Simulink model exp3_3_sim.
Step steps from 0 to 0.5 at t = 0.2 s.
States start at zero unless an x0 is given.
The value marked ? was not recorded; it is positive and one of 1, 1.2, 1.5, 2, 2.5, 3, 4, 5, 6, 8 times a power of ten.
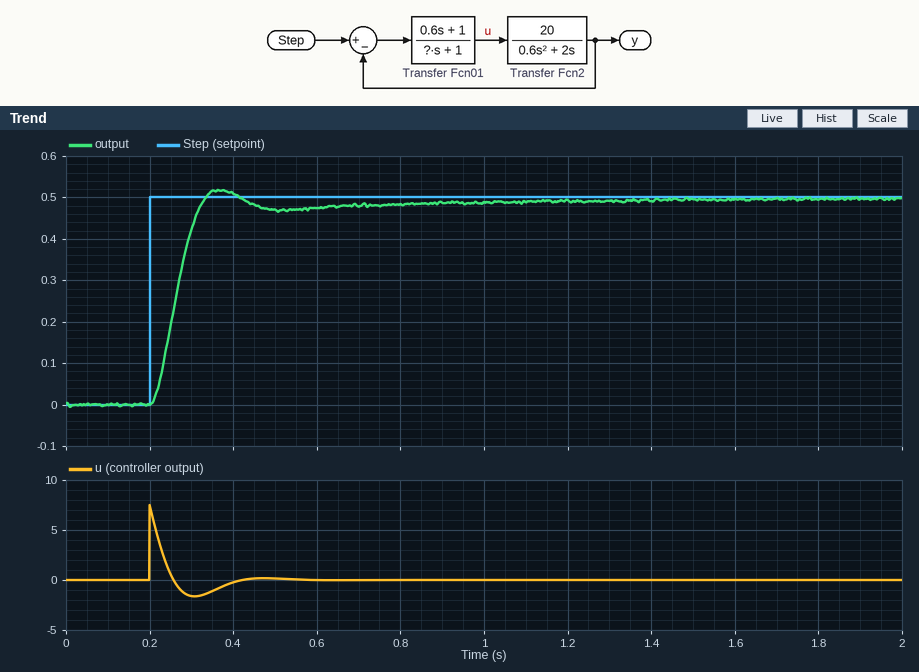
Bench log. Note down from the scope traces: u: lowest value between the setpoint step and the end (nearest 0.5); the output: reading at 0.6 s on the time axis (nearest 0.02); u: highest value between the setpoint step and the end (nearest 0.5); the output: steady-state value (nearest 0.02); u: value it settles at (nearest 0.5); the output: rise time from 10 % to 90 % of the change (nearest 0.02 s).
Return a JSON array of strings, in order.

["-1.5", "0.48", "7.5", "0.50", "0.0", "0.08 s"]
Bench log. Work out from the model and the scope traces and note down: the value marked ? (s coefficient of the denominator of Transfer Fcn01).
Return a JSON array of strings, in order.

["0.04"]
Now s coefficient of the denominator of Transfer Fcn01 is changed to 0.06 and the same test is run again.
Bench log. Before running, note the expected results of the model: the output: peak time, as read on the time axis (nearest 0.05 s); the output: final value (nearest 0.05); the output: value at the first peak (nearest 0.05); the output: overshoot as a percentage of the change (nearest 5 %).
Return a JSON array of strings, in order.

["0.40 s", "0.50", "0.55", "10 %"]
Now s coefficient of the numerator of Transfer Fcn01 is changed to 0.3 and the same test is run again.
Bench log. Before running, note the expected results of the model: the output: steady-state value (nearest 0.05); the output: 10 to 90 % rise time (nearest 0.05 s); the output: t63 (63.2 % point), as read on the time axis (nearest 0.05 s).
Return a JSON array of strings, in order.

["0.50", "0.15 s", "0.30 s"]
